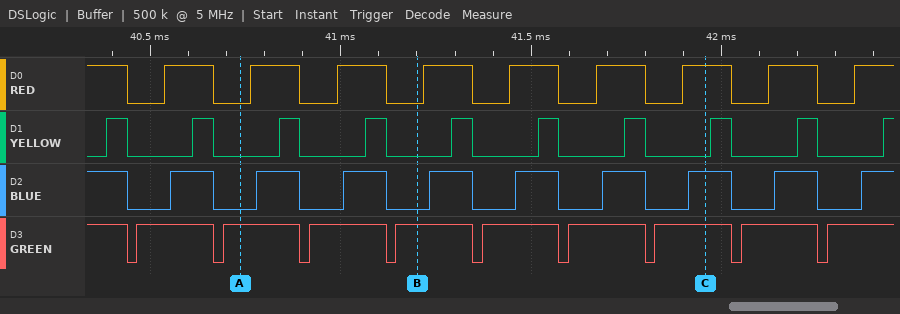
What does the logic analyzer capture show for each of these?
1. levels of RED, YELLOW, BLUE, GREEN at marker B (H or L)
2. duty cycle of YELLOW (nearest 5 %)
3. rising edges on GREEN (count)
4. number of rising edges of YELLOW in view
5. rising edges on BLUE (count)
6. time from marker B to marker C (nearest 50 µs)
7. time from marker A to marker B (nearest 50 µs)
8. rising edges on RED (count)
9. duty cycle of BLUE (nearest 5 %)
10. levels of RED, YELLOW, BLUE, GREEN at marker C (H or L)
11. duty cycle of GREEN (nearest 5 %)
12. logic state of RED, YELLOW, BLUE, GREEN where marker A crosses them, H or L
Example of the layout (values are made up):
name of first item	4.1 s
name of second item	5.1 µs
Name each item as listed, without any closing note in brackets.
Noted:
levels of RED, YELLOW, BLUE, GREEN at marker B	RED=L, YELLOW=L, BLUE=L, GREEN=H
duty cycle of YELLOW	25 %
rising edges on GREEN	9
number of rising edges of YELLOW in view	10
rising edges on BLUE	9
time from marker B to marker C	750 µs
time from marker A to marker B	450 µs
rising edges on RED	9
duty cycle of BLUE	50 %
levels of RED, YELLOW, BLUE, GREEN at marker C	RED=H, YELLOW=L, BLUE=H, GREEN=H
duty cycle of GREEN	90 %
logic state of RED, YELLOW, BLUE, GREEN where marker A crosses them, H or L	RED=L, YELLOW=L, BLUE=L, GREEN=H
